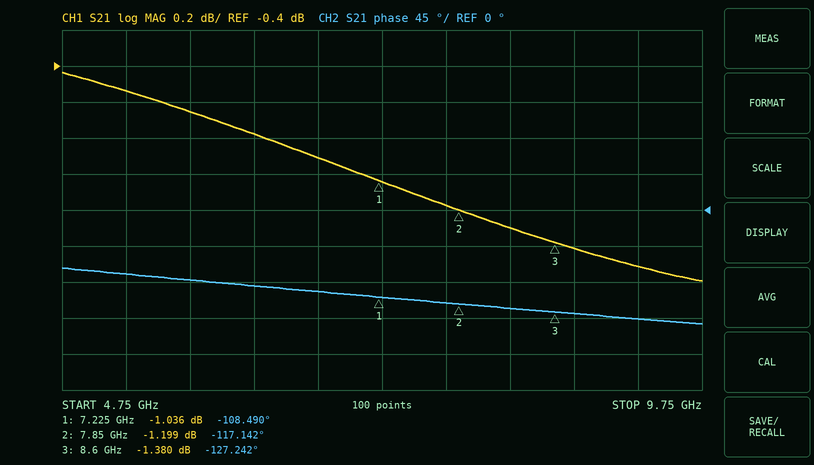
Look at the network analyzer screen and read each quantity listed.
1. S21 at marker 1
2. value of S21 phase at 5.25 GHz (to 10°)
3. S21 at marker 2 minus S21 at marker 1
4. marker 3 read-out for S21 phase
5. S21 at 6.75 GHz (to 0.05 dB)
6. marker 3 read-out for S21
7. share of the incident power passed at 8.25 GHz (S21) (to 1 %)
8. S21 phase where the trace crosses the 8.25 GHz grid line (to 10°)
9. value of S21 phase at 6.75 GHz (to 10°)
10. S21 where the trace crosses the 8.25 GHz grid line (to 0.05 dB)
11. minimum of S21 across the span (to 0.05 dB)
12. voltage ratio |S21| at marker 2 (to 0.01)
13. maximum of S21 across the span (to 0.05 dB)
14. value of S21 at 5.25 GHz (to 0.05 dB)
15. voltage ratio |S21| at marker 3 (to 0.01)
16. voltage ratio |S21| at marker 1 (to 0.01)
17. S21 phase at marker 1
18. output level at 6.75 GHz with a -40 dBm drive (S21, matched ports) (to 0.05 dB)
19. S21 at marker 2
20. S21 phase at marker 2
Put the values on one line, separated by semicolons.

-1.036 dB; -80°; -0.163 dB; -127.242°; -0.90 dB; -1.380 dB; 74 %; -120°; -100°; -1.30 dB; -1.60 dB; 0.87; -0.45 dB; -0.55 dB; 0.85; 0.89; -108.490°; -40.90 dBm; -1.199 dB; -117.142°
